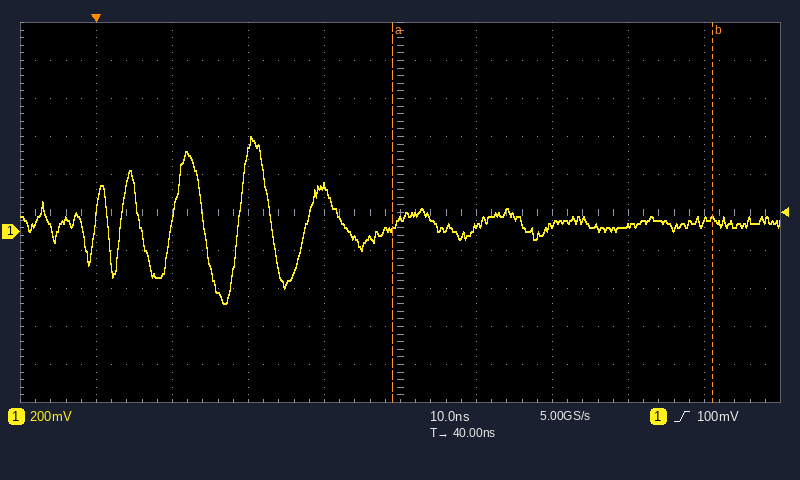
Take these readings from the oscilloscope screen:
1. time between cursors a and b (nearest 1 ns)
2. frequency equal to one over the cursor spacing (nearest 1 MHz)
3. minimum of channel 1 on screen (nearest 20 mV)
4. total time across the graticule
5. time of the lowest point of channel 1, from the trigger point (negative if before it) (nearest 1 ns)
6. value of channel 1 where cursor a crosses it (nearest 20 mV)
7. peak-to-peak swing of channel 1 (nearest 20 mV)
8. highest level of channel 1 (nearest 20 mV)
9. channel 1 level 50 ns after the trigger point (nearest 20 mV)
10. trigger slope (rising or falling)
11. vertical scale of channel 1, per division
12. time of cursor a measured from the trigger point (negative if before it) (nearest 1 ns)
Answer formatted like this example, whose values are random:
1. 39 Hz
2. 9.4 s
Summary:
1. 42 ns
2. 24 MHz
3. -380 mV
4. 100 ns
5. +17 ns
6. 20 mV
7. 880 mV
8. 500 mV
9. 20 mV
10. rising
11. 200 mV
12. +39 ns
